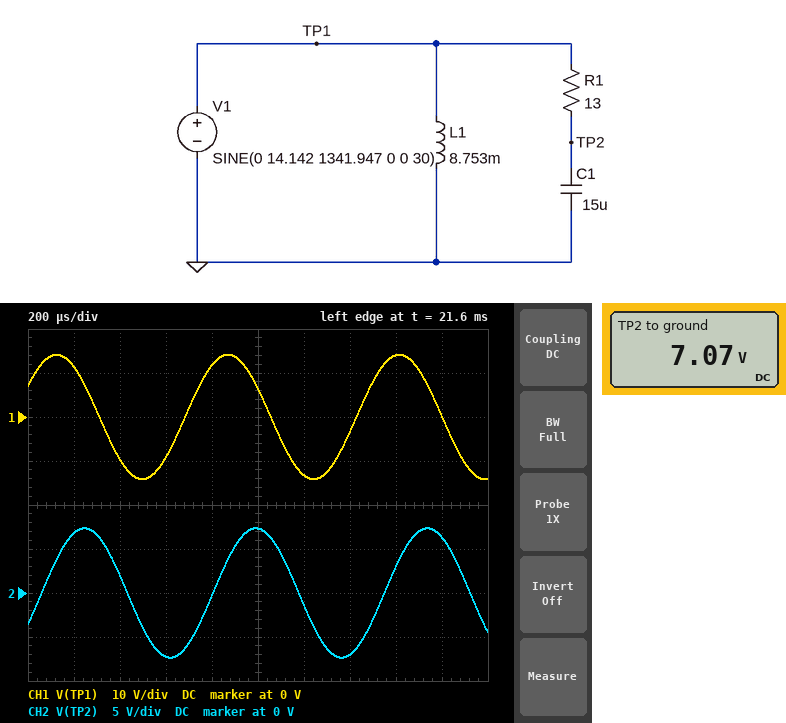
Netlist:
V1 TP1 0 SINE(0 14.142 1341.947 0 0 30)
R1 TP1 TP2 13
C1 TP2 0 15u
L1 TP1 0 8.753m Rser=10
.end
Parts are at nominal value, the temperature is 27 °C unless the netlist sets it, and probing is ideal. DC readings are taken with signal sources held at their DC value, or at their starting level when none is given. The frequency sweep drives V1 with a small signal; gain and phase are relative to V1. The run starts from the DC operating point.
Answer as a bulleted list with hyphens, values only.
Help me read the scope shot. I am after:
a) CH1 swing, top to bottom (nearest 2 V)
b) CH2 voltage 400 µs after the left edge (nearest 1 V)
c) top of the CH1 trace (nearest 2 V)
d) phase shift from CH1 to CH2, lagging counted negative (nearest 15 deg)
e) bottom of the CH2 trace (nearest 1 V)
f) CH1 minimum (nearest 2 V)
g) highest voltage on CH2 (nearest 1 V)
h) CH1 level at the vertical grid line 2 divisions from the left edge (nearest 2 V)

- 28 V
- 2 V
- 14 V
- -60 deg
- -7 V
- -14 V
- 7 V
- -10 V
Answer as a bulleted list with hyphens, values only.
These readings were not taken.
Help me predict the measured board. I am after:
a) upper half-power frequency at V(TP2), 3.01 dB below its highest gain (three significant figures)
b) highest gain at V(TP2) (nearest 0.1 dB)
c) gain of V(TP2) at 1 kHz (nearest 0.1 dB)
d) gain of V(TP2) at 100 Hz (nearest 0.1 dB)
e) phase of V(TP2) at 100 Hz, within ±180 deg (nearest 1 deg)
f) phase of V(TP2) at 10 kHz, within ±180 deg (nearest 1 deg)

- 816 Hz
- 0 dB
- -4.0 dB
- -0.1 dB
- -7 deg
- -85 deg
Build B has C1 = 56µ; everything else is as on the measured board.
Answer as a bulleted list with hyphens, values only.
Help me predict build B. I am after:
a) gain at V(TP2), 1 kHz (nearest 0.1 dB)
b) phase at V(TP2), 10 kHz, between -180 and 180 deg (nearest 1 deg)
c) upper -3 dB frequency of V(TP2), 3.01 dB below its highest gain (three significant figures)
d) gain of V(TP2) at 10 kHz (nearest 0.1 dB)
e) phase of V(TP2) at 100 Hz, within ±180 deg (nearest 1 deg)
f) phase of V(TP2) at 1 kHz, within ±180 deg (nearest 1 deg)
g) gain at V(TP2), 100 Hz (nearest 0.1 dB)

- -13.4 dB
- -89 deg
- 219 Hz
- -33.2 dB
- -25 deg
- -78 deg
- -0.8 dB
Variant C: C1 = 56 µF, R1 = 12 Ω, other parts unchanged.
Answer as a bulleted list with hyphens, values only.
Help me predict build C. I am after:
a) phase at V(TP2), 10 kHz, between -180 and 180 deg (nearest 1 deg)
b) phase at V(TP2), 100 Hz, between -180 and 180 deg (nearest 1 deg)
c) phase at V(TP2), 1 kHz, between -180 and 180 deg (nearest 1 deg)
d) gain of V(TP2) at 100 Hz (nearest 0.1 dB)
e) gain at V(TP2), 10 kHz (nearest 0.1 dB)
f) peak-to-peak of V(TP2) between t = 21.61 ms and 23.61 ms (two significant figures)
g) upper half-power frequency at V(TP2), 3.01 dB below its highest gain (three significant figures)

- -89 deg
- -23 deg
- -77 deg
- -0.7 dB
- -32.5 dB
- 4.9 V
- 237 Hz
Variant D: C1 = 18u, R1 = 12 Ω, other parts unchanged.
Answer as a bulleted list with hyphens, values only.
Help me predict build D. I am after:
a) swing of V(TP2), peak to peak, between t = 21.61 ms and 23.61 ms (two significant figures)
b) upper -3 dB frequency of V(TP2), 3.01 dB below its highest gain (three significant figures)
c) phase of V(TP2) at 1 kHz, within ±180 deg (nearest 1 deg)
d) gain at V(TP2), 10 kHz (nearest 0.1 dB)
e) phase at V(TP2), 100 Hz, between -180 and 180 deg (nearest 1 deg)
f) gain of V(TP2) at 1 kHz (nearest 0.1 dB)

- 14 V
- 737 Hz
- -54 deg
- -22.7 dB
- -8 deg
- -4.5 dB
